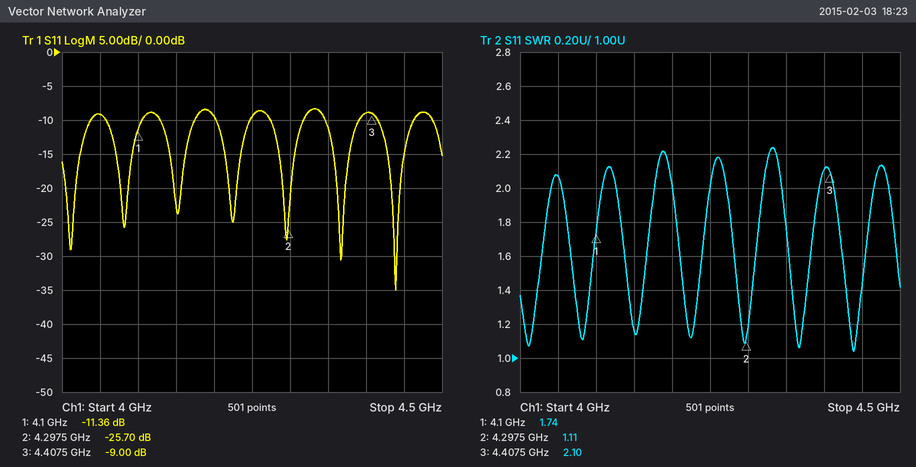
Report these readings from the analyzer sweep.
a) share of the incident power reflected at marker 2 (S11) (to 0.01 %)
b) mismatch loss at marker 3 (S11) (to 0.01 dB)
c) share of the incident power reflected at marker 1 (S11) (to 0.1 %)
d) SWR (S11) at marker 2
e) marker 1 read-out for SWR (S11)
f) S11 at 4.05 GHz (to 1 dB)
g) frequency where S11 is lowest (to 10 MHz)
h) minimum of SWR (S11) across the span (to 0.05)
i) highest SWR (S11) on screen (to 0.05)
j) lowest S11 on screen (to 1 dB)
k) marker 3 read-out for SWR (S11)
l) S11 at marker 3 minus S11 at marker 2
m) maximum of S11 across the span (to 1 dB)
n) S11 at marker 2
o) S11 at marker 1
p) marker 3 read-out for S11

0.27 %
0.58 dB
7.3 %
1.11
1.74
-9 dB
4.44 GHz
1.05
2.25
-35 dB
2.10
16.70 dB
-8 dB
-25.70 dB
-11.36 dB
-9.00 dB
